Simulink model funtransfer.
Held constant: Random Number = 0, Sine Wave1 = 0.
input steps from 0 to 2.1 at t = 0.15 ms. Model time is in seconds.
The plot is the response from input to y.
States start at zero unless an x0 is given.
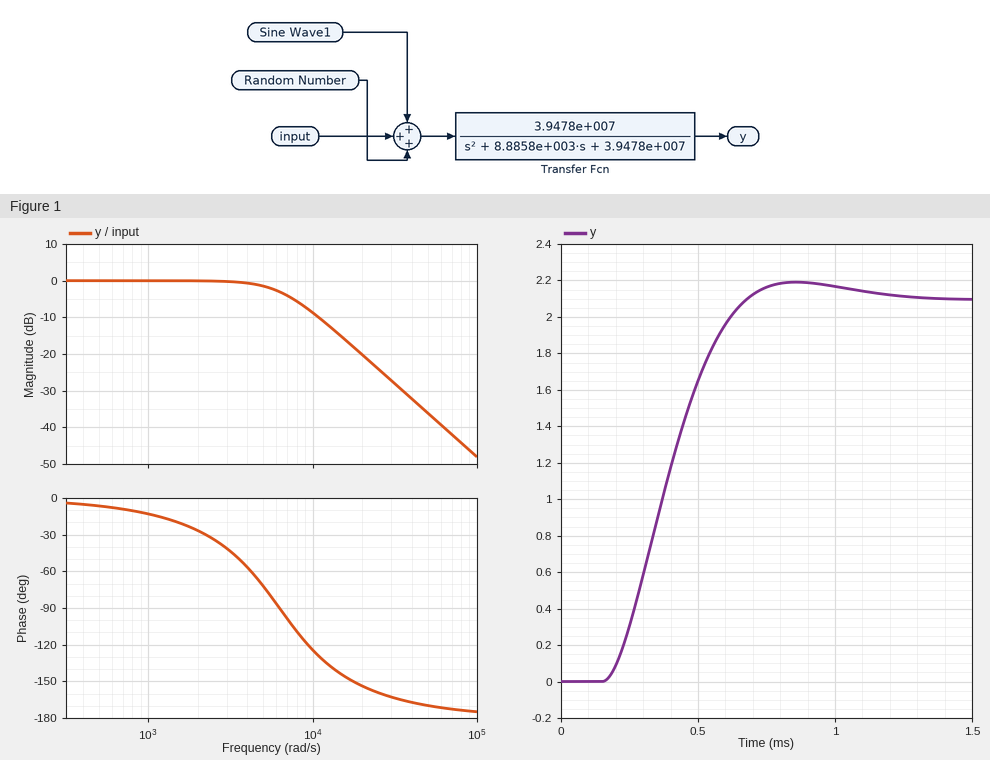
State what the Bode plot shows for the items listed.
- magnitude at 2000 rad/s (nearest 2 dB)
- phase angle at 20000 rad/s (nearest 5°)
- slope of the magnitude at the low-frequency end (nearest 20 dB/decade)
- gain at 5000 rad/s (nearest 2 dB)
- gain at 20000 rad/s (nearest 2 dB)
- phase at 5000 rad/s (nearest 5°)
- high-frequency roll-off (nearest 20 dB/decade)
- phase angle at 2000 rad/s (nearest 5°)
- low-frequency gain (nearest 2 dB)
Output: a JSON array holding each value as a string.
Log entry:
["0 dB", "-155°", "0 dB/decade", "-2 dB", "-20 dB", "-70°", "-40 dB/decade", "-25°", "0 dB"]
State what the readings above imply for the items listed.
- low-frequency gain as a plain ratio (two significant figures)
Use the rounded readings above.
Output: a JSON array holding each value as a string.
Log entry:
["1.0"]
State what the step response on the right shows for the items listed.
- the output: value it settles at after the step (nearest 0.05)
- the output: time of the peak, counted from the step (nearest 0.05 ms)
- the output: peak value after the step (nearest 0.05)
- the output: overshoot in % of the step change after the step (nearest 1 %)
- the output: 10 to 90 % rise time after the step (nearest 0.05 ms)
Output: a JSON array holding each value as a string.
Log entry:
["2.10", "0.70 ms", "2.20", "4 %", "0.35 ms"]
